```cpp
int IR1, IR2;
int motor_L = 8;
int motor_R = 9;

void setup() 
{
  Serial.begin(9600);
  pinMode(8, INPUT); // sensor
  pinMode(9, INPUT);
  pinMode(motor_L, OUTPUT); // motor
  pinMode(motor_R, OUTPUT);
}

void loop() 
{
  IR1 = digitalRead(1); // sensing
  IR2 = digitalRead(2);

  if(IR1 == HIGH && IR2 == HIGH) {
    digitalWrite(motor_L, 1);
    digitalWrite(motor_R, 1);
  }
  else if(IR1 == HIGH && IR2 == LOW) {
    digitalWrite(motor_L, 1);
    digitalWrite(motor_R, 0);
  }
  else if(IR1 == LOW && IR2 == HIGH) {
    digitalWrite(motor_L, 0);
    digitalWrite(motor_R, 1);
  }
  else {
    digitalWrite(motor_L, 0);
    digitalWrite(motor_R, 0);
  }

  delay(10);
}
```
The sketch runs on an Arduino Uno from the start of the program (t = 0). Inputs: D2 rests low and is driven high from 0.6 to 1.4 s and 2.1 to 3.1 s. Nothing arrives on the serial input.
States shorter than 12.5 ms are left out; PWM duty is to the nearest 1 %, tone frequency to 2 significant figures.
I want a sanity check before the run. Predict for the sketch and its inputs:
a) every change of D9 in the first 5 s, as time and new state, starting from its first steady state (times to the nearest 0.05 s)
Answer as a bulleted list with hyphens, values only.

- 0 s low; 0.6 s high; 1.4 s low; 2.1 s high; 3.1 s low
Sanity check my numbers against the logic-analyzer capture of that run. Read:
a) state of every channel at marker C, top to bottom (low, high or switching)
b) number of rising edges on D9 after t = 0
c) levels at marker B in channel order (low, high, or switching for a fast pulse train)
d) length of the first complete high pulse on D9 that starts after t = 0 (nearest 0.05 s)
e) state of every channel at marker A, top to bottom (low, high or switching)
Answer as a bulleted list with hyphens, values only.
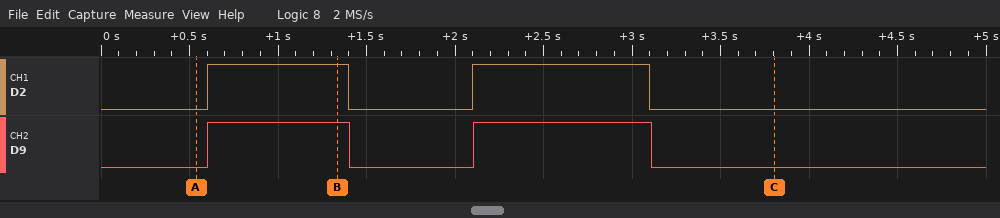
- D2 low, D9 low
- 2
- D2 high, D9 high
- 0.80 s
- D2 low, D9 low
